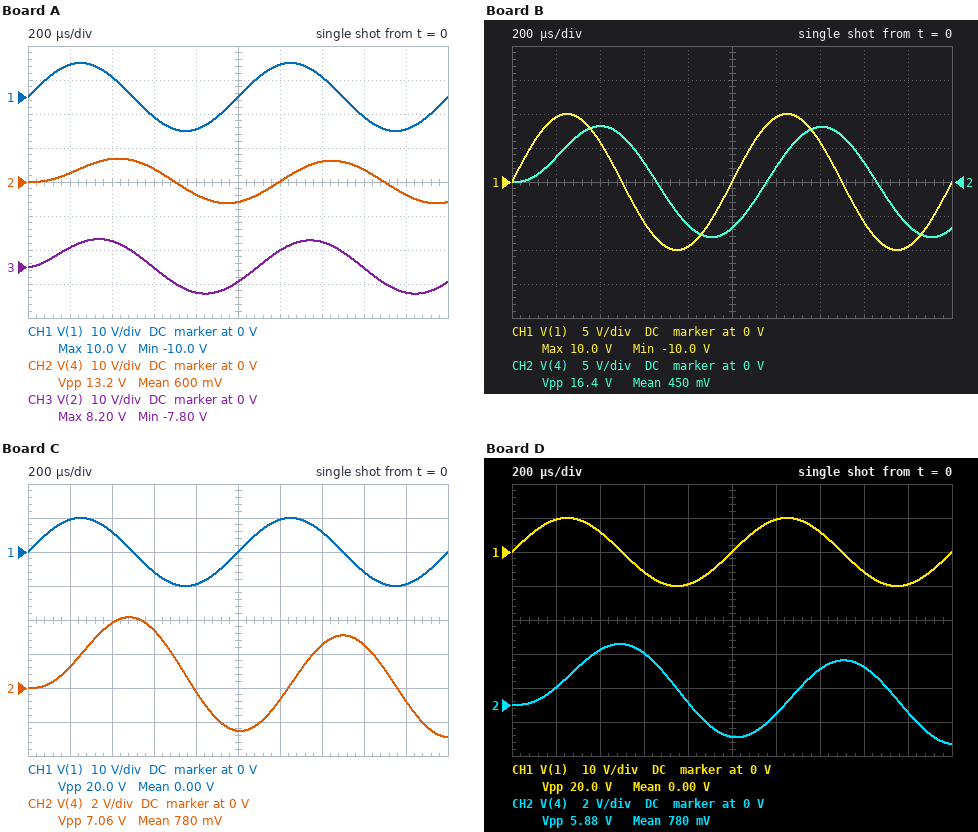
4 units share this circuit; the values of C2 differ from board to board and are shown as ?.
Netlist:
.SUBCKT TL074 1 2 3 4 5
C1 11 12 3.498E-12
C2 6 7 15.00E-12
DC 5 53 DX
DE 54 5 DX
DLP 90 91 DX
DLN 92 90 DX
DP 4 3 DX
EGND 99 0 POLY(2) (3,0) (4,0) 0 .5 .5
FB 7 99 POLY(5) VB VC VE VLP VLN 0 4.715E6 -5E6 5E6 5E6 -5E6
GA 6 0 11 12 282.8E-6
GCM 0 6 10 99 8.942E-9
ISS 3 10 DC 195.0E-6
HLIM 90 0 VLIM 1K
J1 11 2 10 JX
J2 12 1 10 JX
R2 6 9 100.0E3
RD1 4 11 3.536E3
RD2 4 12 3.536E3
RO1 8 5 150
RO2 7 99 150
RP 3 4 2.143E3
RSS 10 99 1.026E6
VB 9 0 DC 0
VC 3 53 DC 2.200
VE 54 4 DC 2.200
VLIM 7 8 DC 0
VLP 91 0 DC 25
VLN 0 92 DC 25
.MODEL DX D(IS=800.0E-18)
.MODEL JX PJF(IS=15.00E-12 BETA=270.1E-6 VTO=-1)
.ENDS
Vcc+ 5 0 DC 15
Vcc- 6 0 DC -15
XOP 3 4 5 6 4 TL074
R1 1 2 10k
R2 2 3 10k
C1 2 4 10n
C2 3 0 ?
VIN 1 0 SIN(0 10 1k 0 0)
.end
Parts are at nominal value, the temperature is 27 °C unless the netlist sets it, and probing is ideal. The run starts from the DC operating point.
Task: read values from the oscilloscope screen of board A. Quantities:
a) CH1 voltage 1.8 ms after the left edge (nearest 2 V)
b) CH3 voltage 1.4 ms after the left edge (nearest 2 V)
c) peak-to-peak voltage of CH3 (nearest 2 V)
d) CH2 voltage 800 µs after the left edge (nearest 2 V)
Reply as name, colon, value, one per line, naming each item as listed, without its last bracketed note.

CH1 voltage 1.8 ms after the left edge: -10 V
CH3 voltage 1.4 ms after the left edge: 8 V
peak-to-peak voltage of CH3: 16 V
CH2 voltage 800 µs after the left edge: -4 V
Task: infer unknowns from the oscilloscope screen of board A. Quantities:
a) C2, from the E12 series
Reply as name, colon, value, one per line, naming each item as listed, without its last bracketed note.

C2, from the E12 series: 12 nF
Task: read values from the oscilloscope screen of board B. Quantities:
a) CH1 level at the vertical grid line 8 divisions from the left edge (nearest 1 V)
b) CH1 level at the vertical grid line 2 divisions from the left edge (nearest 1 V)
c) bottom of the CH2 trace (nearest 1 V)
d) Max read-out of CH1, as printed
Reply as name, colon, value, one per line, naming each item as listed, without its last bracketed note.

CH1 level at the vertical grid line 8 divisions from the left edge: -6 V
CH1 level at the vertical grid line 2 divisions from the left edge: 6 V
bottom of the CH2 trace: -8 V
Max read-out of CH1, as printed: 10.0 V
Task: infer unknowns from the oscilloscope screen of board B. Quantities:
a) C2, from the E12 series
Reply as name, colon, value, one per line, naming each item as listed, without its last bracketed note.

C2, from the E12 series: 8.2 nF
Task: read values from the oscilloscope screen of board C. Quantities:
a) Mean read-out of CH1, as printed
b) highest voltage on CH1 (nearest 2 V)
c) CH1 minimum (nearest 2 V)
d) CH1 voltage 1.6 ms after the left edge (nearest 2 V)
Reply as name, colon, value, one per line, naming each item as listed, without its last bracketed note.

Mean read-out of CH1, as printed: 0.00 V
highest voltage on CH1: 10 V
CH1 minimum: -10 V
CH1 voltage 1.6 ms after the left edge: -6 V
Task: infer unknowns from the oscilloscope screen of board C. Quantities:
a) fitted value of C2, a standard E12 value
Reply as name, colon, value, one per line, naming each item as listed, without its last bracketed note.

fitted value of C2, a standard E12 value: 27 nF
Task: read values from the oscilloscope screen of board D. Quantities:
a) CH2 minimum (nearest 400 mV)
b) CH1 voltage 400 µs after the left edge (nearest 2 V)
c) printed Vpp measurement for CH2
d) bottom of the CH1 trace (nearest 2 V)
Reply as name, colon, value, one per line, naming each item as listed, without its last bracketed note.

CH2 minimum: -2.4 V
CH1 voltage 400 µs after the left edge: 6 V
printed Vpp measurement for CH2: 5.88 V
bottom of the CH1 trace: -10 V
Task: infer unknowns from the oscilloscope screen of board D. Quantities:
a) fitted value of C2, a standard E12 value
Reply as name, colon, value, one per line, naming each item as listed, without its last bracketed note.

fitted value of C2, a standard E12 value: 33 nF
